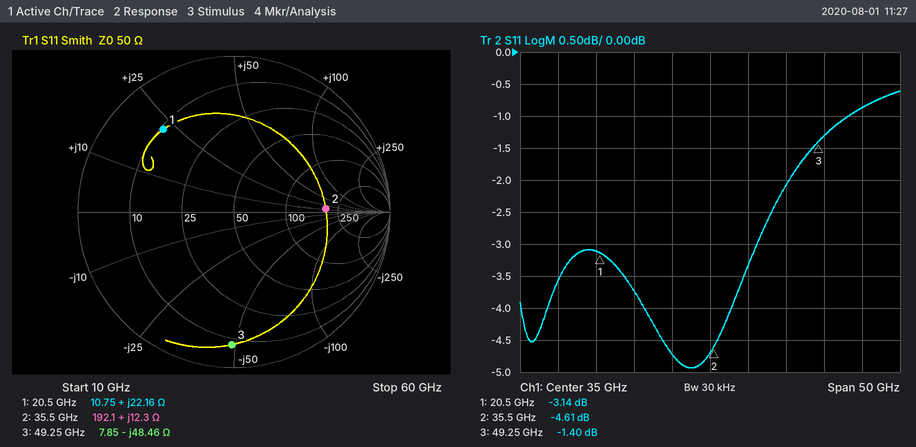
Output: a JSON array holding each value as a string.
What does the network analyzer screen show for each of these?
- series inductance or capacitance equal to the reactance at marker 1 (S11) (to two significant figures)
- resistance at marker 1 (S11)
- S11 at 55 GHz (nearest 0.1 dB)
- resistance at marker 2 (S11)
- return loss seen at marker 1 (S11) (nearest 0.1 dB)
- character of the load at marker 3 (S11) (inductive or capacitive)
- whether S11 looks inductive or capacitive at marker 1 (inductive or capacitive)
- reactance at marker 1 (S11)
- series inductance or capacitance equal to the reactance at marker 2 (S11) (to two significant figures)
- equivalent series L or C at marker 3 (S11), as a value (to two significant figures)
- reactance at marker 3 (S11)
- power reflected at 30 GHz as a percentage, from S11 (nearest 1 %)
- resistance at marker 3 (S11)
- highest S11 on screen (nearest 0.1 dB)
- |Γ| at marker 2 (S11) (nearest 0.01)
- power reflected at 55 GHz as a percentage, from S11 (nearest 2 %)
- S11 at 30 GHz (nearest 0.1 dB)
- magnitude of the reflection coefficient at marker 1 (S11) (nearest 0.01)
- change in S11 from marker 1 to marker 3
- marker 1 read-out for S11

["170 pH", "10.75 Ω", "-0.9 dB", "192.1 Ω", "3.1 dB", "capacitive", "inductive", "+22.16 Ω", "55 pH", "67 fF", "-48.46 Ω", "34 %", "7.85 Ω", "-0.6 dB", "0.59", "82 %", "-4.7 dB", "0.70", "1.74 dB", "-3.14 dB"]
